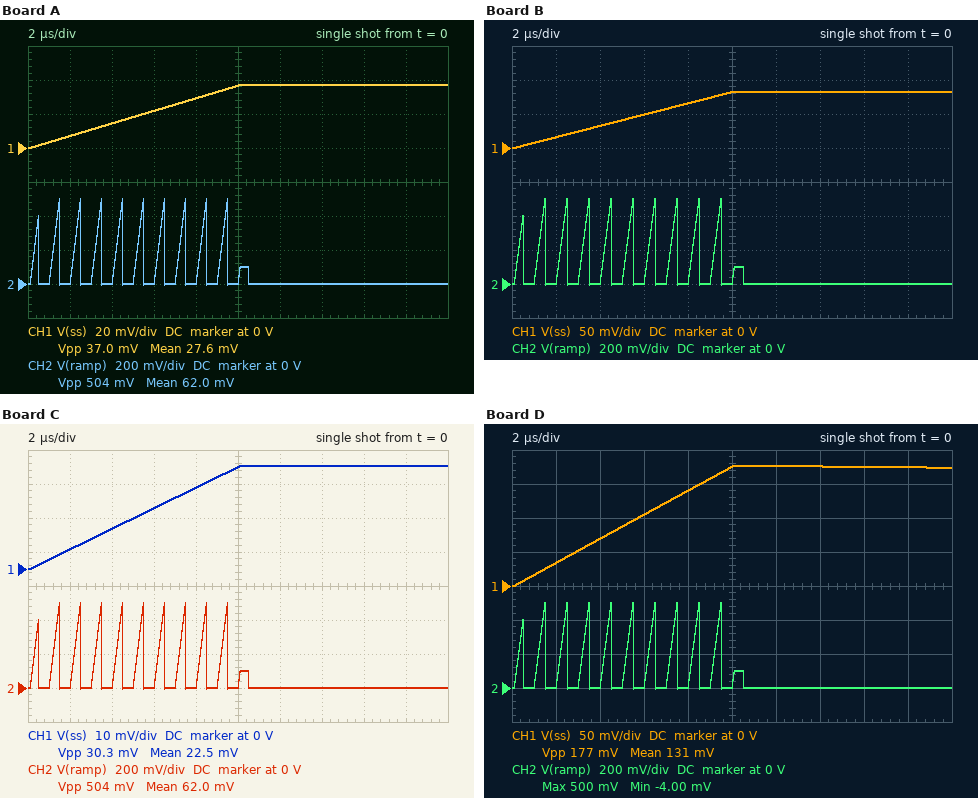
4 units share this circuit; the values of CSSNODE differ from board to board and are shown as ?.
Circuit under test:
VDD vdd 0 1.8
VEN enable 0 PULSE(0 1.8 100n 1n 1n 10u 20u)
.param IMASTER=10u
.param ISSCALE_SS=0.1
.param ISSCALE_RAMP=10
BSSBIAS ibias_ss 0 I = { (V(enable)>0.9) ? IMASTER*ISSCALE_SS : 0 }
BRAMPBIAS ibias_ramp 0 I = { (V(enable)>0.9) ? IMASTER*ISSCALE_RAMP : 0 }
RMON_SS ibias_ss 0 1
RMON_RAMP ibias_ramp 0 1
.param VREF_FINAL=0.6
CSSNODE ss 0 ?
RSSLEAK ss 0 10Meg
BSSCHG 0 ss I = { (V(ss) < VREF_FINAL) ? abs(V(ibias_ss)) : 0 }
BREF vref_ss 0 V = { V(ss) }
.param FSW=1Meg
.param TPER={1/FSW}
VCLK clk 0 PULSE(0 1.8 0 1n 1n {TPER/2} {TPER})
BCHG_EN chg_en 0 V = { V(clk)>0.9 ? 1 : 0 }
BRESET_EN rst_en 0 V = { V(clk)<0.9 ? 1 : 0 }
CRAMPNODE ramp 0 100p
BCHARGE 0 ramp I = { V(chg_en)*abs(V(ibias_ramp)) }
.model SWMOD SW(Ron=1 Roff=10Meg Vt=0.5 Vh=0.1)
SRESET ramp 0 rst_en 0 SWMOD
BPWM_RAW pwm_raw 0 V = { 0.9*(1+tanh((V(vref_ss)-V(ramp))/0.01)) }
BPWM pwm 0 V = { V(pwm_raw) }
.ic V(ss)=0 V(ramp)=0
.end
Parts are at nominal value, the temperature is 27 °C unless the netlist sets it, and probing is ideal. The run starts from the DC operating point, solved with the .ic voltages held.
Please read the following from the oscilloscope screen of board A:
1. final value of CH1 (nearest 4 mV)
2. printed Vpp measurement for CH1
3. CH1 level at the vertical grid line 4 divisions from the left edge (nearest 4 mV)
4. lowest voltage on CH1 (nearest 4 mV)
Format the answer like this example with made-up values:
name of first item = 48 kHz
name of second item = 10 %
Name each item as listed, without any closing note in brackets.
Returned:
final value of CH1 = 36 mV
printed Vpp measurement for CH1 = 37.0 mV
CH1 level at the vertical grid line 4 divisions from the left edge = 28 mV
lowest voltage on CH1 = 0 V
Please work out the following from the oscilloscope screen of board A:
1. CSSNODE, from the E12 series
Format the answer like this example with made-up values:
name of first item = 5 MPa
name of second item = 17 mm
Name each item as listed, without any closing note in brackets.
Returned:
CSSNODE, from the E12 series = 270 pF
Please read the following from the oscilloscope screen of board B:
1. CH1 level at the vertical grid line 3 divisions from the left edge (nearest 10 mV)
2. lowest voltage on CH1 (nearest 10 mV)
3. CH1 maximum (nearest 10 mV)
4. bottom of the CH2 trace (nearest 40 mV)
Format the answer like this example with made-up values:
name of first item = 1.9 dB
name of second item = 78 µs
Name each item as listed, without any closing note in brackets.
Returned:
CH1 level at the vertical grid line 3 divisions from the left edge = 50 mV
lowest voltage on CH1 = 0 V
CH1 maximum = 80 mV
bottom of the CH2 trace = 0 V
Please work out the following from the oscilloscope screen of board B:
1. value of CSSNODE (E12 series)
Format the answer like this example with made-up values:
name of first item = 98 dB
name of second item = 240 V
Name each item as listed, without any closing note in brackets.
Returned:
value of CSSNODE = 120 pF
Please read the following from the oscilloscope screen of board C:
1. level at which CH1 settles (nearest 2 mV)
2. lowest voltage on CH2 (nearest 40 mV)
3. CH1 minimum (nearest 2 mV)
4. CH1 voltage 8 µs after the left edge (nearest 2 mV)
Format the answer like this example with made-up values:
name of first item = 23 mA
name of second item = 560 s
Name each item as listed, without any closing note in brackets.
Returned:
level at which CH1 settles = 30 mV
lowest voltage on CH2 = 0 V
CH1 minimum = 0 V
CH1 voltage 8 µs after the left edge = 24 mV
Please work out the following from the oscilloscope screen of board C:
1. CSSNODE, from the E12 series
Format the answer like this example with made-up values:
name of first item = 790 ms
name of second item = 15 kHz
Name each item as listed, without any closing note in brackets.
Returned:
CSSNODE, from the E12 series = 330 pF
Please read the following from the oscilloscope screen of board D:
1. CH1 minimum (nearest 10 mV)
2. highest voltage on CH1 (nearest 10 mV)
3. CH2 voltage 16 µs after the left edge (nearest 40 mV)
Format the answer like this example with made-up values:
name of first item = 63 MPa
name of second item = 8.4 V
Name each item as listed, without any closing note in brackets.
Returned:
CH1 minimum = 0 V
highest voltage on CH1 = 180 mV
CH2 voltage 16 µs after the left edge = 0 V
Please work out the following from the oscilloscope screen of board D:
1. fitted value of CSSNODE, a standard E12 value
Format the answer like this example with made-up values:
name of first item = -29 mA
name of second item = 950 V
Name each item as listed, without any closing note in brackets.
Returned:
fitted value of CSSNODE, a standard E12 value = 56 pF
